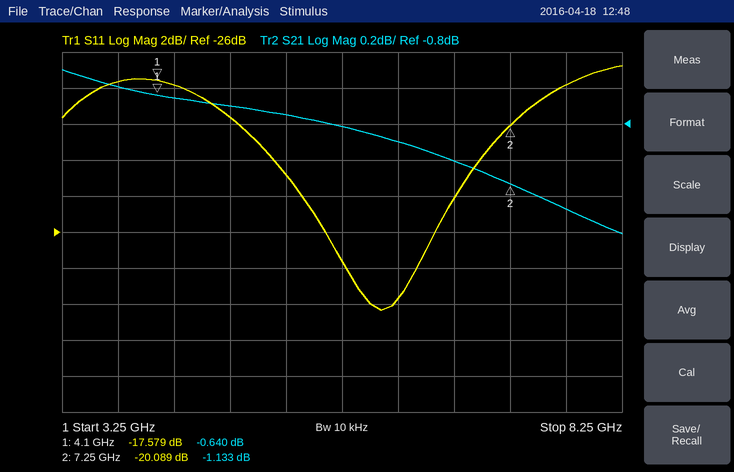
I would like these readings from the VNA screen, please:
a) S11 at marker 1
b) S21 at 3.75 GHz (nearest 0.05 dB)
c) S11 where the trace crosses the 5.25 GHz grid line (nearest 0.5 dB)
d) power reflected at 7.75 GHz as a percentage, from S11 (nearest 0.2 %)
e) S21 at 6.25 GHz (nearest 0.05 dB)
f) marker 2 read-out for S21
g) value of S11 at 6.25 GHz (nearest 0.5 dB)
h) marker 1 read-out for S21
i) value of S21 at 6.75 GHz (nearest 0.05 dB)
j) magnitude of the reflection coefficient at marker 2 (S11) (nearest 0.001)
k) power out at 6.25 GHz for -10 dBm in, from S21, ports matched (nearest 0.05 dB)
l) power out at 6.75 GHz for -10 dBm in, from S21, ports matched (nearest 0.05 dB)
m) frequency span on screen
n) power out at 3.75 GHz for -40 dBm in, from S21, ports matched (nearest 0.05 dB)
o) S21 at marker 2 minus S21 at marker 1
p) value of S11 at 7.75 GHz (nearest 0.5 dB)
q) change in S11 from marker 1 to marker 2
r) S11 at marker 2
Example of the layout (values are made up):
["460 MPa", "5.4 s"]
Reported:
["-17.579 dB", "-0.60 dB", "-23.0 dB", "1.6 %", "-0.90 dB", "-1.133 dB", "-29.5 dB", "-0.640 dB", "-1.00 dB", "0.099", "-10.90 dBm", "-11.00 dBm", "5 GHz", "-40.60 dBm", "-0.493 dB", "-18.0 dB", "-2.510 dB", "-20.089 dB"]
